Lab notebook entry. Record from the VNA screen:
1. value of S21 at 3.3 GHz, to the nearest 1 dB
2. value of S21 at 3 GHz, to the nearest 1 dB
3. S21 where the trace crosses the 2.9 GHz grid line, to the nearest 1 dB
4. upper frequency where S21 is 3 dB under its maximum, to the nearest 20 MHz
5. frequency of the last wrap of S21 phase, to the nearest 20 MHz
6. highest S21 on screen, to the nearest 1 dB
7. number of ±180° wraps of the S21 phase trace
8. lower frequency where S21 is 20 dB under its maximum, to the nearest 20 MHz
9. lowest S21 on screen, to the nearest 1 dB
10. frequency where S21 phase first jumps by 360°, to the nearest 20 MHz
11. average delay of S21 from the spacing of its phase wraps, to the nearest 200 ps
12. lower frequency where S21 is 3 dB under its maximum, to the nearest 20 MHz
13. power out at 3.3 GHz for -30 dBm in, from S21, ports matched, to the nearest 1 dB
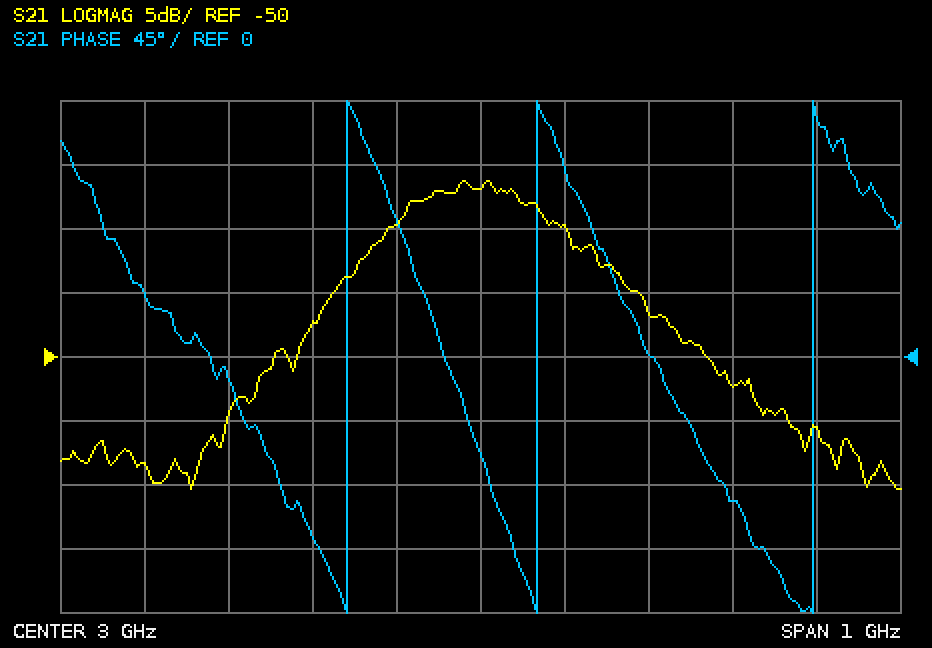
-52 dB
-37 dB
-40 dB
3.08 GHz
3.40 GHz
-36 dB
3
2.70 GHz
-60 dB
2.84 GHz
3.6 ns
2.90 GHz
-82 dBm
